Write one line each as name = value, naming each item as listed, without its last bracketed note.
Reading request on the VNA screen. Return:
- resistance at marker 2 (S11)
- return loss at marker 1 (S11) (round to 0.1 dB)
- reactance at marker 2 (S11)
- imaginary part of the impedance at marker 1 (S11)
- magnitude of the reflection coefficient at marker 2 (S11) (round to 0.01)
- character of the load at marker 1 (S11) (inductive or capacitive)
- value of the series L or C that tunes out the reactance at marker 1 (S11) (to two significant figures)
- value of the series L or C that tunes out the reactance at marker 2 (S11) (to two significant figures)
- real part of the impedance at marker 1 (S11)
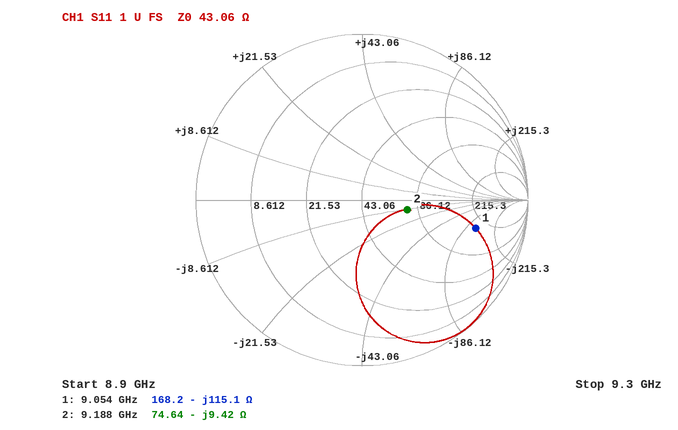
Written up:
resistance at marker 2 = 74.64 Ω
return loss at marker 1 (S11) = 3.0 dB
reactance at marker 2 = -9.42 Ω
imaginary part of the impedance at marker 1 = -115.1 Ω
magnitude of the reflection coefficient at marker 2 (S11) = 0.28
character of the load at marker 1 (S11) = capacitive
value of the series L or C that tunes out the reactance at marker 1 (S11) = 2.0 nH
value of the series L or C that tunes out the reactance at marker 2 (S11) = 160 pH
real part of the impedance at marker 1 = 168.2 Ω
